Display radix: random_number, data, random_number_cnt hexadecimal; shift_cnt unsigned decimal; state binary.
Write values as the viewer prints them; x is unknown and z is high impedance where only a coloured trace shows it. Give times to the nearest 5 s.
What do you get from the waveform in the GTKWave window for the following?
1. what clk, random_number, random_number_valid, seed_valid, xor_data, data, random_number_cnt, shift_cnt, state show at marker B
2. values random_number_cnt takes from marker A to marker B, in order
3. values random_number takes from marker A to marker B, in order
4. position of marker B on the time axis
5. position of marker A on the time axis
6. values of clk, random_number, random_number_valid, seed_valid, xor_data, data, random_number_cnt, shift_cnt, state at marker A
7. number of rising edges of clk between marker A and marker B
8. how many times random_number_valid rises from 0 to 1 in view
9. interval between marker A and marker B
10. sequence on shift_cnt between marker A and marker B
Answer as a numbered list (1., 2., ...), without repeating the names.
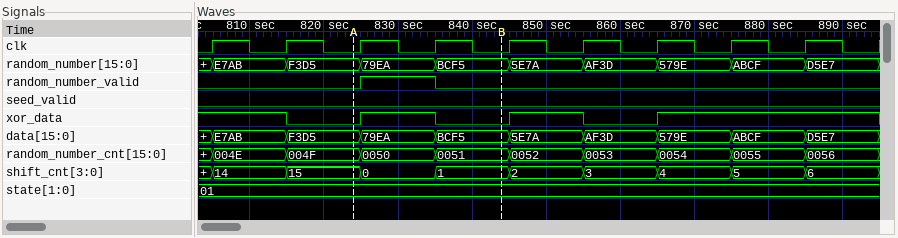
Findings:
1. clk=0, random_number=BCF5, random_number_valid=0, seed_valid=0, xor_data=0, data=BCF5, random_number_cnt=0051, shift_cnt=1, state=01
2. 004F, 0050, 0051
3. F3D5, 79EA, BCF5
4. 845 s
5. 825 s
6. clk=0, random_number=F3D5, random_number_valid=0, seed_valid=0, xor_data=0, data=F3D5, random_number_cnt=004F, shift_cnt=15, state=01
7. 2
8. 1
9. 20 s
10. 15, 0, 1
